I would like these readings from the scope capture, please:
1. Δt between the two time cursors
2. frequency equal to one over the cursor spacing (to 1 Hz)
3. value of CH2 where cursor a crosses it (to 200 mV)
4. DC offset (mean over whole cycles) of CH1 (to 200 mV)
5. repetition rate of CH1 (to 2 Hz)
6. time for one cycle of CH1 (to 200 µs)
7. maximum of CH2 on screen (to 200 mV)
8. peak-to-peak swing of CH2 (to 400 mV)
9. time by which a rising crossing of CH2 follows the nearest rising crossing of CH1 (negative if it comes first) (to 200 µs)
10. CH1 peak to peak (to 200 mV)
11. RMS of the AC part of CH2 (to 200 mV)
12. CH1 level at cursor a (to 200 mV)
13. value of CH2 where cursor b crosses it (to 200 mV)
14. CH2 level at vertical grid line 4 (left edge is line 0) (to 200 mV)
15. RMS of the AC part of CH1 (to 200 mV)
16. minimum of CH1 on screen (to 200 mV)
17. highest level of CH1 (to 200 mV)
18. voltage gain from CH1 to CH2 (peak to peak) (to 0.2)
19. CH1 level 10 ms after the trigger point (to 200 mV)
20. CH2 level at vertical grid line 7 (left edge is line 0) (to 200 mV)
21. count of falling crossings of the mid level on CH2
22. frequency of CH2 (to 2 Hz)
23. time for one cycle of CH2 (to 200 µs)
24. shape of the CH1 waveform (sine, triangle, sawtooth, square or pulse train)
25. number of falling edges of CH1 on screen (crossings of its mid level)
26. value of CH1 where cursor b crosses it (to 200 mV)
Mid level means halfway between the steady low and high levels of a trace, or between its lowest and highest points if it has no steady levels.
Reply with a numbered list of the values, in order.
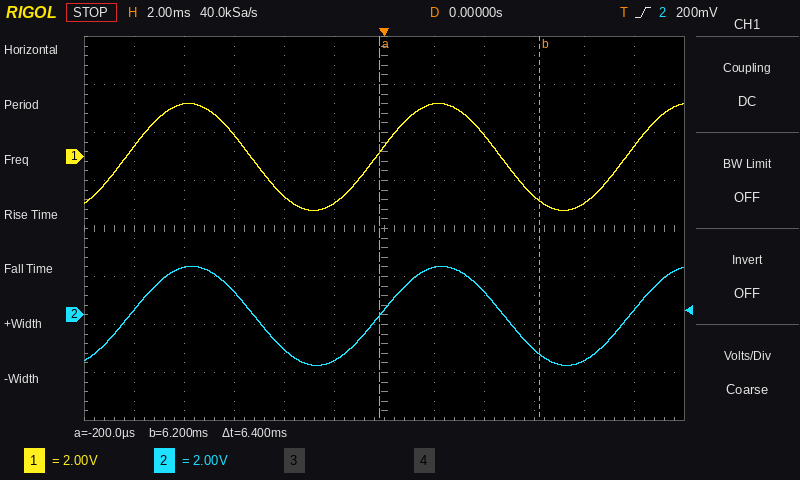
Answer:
1. 6.4 ms
2. 156 Hz
3. 0.0 V
4. 0.0 V
5. 100 Hz
6. 10.0 ms
7. 2.0 V
8. 4.0 V
9. +200 µs
10. 4.4 V
11. 1.4 V
12. 200 mV
13. -1.6 V
14. -1.4 V
15. 1.6 V
16. -2.2 V
17. 2.2 V
18. 1.0
19. 400 mV
20. 2.0 V
21. 2
22. 100 Hz
23. 10.0 ms
24. sine
25. 2
26. -1.8 V
